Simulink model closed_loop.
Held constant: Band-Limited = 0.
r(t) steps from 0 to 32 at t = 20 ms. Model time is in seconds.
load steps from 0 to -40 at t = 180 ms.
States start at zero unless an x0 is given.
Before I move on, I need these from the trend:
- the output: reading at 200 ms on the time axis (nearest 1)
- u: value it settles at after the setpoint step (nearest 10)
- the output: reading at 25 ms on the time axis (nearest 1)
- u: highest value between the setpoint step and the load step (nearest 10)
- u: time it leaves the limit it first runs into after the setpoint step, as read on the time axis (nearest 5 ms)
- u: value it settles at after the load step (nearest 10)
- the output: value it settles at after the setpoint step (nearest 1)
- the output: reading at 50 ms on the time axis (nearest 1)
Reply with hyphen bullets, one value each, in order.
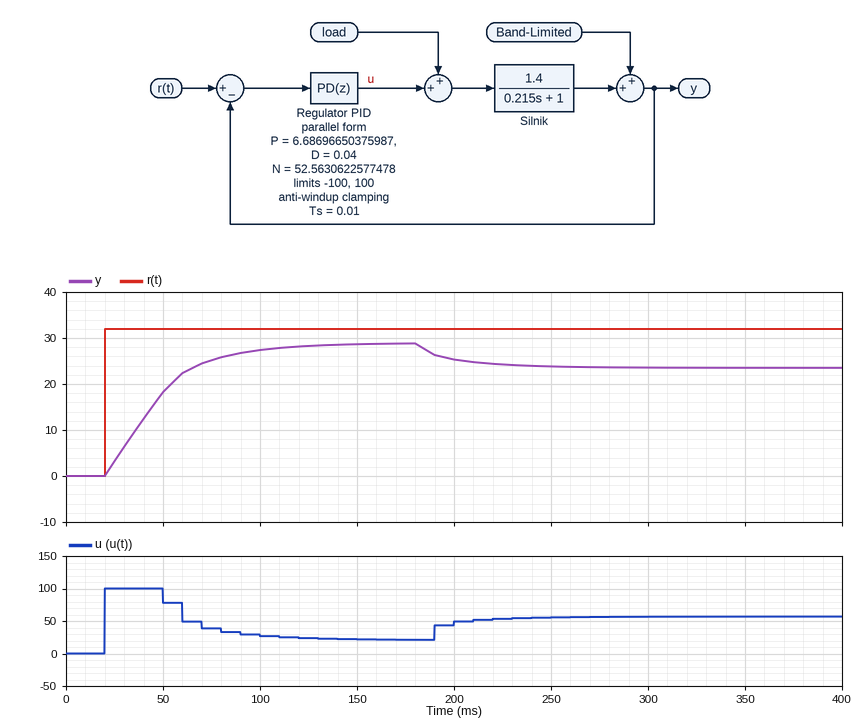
- 25
- 20
- 3
- 100
- 50 ms
- 60
- 29
- 18
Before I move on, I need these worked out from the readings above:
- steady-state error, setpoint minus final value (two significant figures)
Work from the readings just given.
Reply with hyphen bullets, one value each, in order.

- 3.0
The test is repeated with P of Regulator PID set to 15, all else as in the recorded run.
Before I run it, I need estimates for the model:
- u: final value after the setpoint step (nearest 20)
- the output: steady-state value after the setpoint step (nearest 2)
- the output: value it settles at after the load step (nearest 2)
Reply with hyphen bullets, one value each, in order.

- 20
- 30
- 28
